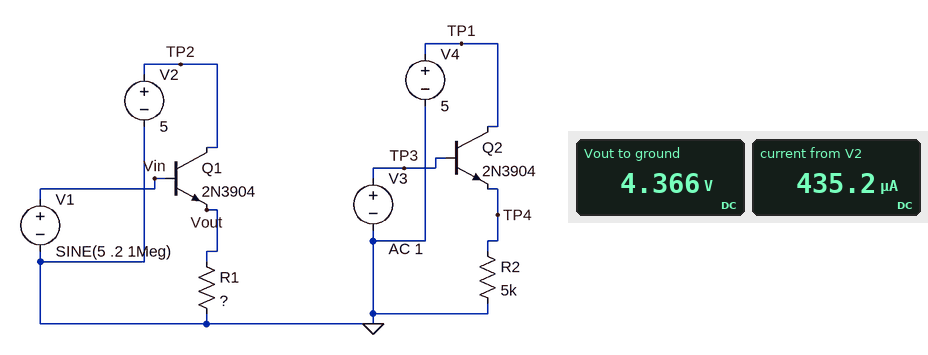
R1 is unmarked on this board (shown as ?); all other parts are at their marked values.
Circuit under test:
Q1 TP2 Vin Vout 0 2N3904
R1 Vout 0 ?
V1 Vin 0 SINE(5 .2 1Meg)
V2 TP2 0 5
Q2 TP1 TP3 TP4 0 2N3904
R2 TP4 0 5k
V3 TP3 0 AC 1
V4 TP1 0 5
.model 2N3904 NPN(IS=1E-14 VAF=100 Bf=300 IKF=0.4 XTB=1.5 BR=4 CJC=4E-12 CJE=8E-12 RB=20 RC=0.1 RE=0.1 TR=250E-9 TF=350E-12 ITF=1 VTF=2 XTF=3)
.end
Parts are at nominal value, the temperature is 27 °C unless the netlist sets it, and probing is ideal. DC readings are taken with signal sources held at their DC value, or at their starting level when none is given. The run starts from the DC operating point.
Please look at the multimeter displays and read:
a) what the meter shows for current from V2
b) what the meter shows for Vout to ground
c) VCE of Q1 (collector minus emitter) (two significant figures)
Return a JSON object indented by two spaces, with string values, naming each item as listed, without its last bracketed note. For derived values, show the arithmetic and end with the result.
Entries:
{
  "what the meter shows for current from V2": "435.2 µA",
  "what the meter shows for Vout to ground": "4.366 V",
  "VCE of Q1 (collector minus emitter)": "5 V - 4.366 V = 630 mV"
}
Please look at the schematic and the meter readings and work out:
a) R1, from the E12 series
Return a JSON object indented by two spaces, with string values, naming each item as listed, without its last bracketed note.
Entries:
{
  "R1, from the E12 series": "10 kΩ"
}
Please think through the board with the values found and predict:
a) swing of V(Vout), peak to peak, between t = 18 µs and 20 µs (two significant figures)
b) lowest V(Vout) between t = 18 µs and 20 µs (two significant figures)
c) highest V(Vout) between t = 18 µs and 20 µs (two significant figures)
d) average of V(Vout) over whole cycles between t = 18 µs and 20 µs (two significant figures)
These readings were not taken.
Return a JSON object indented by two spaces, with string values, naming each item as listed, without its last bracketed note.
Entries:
{
  "swing of V(Vout), peak to peak, between t = 18 µs and 20 µs": "400 mV",
  "lowest V(Vout) between t = 18 µs and 20 µs": "4.2 V",
  "highest V(Vout) between t = 18 µs and 20 µs": "4.6 V",
  "average of V(Vout) over whole cycles between t = 18 µs and 20 µs": "4.4 V"
}
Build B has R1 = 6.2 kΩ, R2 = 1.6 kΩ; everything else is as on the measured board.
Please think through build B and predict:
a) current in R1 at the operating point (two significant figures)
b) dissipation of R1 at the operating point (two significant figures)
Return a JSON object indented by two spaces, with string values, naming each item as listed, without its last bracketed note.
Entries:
{
  "current in R1 at the operating point": "700 µA",
  "dissipation of R1 at the operating point": "3.1 mW"
}
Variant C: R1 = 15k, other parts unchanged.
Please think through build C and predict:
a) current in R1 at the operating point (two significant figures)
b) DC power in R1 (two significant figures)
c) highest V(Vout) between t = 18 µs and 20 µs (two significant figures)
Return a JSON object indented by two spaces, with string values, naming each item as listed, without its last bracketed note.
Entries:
{
  "current in R1 at the operating point": "290 µA",
  "DC power in R1": "1.3 mW",
  "highest V(Vout) between t = 18 µs and 20 µs": "4.6 V"
}
